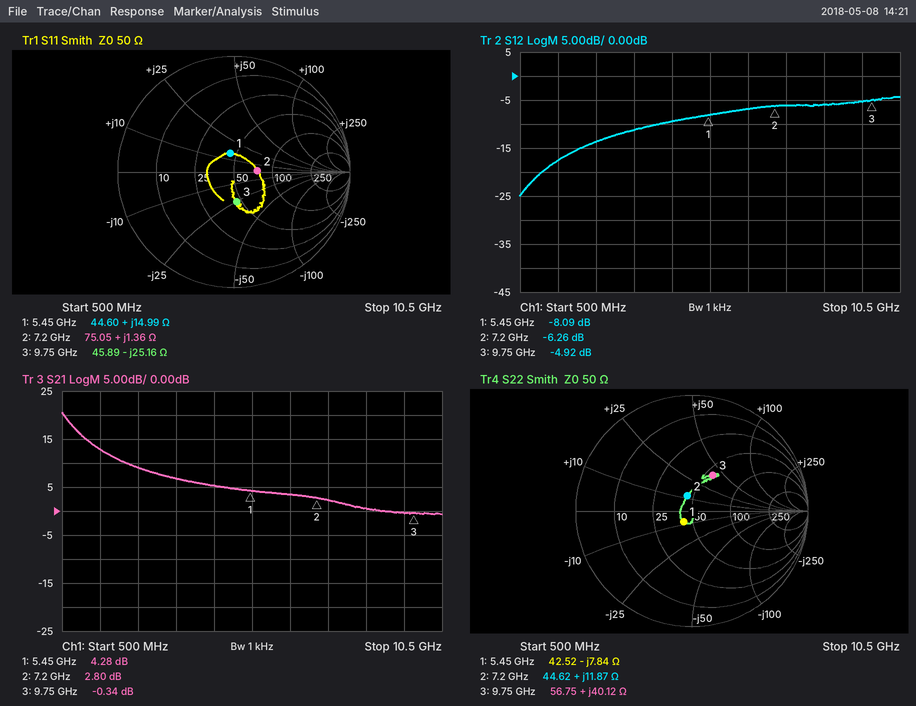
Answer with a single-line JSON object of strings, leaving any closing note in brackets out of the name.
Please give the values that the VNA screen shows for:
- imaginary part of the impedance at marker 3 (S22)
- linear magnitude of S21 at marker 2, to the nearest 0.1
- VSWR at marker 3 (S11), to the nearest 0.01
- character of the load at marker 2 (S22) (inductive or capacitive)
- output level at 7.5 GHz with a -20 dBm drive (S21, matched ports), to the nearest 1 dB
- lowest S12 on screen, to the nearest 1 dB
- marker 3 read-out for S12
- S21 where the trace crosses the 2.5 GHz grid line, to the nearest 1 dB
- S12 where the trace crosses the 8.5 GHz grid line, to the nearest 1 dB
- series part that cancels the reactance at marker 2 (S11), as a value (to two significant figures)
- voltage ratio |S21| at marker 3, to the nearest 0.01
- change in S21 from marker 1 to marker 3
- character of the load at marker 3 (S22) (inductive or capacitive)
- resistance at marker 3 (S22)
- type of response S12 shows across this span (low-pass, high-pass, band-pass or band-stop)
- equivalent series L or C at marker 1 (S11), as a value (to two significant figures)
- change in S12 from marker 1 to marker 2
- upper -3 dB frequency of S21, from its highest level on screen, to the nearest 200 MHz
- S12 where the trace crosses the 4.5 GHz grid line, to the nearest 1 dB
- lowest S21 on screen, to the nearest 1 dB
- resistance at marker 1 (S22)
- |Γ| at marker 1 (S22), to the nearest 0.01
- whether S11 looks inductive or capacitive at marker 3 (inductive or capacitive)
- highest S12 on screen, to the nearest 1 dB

{"imaginary part of the impedance at marker 3": "+40.12 Ω", "linear magnitude of S21 at marker 2, to the nearest 0.1": "1.4", "VSWR at marker 3 (S11), to the nearest 0.01": "1.69", "character of the load at marker 2 (S22)": "inductive", "output level at 7.5 GHz with a -20 dBm drive (S21, matched ports), to the nearest 1 dB": "-18 dBm", "lowest S12 on screen, to the nearest 1 dB": "-25 dB", "marker 3 read-out for S12": "-4.92 dB", "S21 where the trace crosses the 2.5 GHz grid line, to the nearest 1 dB": "9 dB", "S12 where the trace crosses the 8.5 GHz grid line, to the nearest 1 dB": "-6 dB", "series part that cancels the reactance at marker 2 (S11), as a value": "16 pF", "voltage ratio |S21| at marker 3, to the nearest 0.01": "0.96", "change in S21 from marker 1 to marker 3": "-4.62 dB", "character of the load at marker 3 (S22)": "inductive", "resistance at marker 3": "56.75 Ω", "type of response S12 shows across this span": "high-pass", "equivalent series L or C at marker 1 (S11), as a value": "440 pH", "change in S12 from marker 1 to marker 2": "1.83 dB", "upper -3 dB frequency of S21, from its highest level on screen, to the nearest 200 MHz": "800 MHz", "S12 where the trace crosses the 4.5 GHz grid line, to the nearest 1 dB": "-9 dB", "lowest S21 on screen, to the nearest 1 dB": "-1 dB", "resistance at marker 1": "42.52 Ω", "|Γ| at marker 1 (S22), to the nearest 0.01": "0.12", "whether S11 looks inductive or capacitive at marker 3": "capacitive", "highest S12 on screen, to the nearest 1 dB": "-4 dB"}
